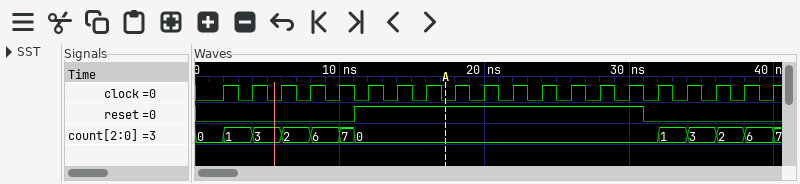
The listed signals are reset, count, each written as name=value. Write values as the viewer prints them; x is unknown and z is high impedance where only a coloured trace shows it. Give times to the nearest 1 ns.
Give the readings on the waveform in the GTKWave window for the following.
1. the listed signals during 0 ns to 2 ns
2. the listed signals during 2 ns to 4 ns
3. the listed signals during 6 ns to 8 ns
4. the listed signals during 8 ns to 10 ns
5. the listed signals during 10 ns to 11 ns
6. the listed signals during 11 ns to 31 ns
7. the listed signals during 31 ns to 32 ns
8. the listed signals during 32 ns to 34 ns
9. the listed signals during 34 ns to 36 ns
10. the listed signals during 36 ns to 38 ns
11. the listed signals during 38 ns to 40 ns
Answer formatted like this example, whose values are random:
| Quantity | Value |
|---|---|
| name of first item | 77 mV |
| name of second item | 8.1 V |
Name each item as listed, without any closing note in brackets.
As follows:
| Quantity | Value |
|---|---|
| the listed signals during 0 ns to 2 ns | reset=0, count=0 |
| the listed signals during 2 ns to 4 ns | reset=0, count=1 |
| the listed signals during 6 ns to 8 ns | reset=0, count=2 |
| the listed signals during 8 ns to 10 ns | reset=0, count=6 |
| the listed signals during 10 ns to 11 ns | reset=0, count=7 |
| the listed signals during 11 ns to 31 ns | reset=1, count=0 |
| the listed signals during 31 ns to 32 ns | reset=0, count=0 |
| the listed signals during 32 ns to 34 ns | reset=0, count=1 |
| the listed signals during 34 ns to 36 ns | reset=0, count=3 |
| the listed signals during 36 ns to 38 ns | reset=0, count=2 |
| the listed signals during 38 ns to 40 ns | reset=0, count=6 |
